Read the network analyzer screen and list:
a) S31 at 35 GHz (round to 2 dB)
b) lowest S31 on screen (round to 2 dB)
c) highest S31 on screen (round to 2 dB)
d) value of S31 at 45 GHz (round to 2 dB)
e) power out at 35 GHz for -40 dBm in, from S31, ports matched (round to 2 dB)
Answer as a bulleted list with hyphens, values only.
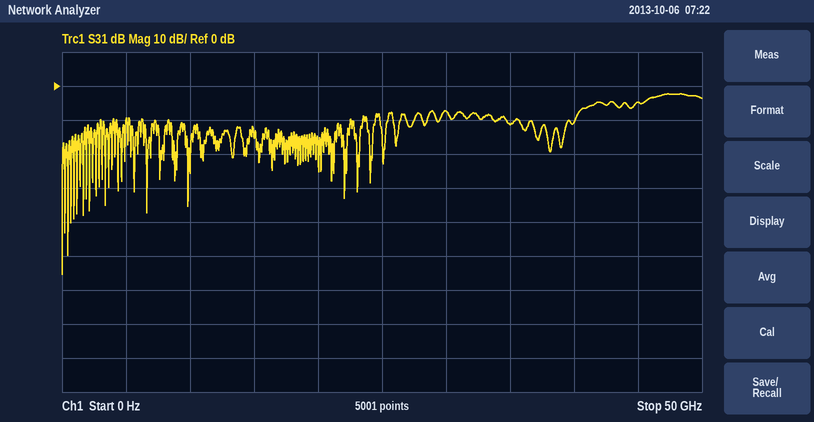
- -12 dB
- -56 dB
- -2 dB
- -4 dB
- -52 dBm
